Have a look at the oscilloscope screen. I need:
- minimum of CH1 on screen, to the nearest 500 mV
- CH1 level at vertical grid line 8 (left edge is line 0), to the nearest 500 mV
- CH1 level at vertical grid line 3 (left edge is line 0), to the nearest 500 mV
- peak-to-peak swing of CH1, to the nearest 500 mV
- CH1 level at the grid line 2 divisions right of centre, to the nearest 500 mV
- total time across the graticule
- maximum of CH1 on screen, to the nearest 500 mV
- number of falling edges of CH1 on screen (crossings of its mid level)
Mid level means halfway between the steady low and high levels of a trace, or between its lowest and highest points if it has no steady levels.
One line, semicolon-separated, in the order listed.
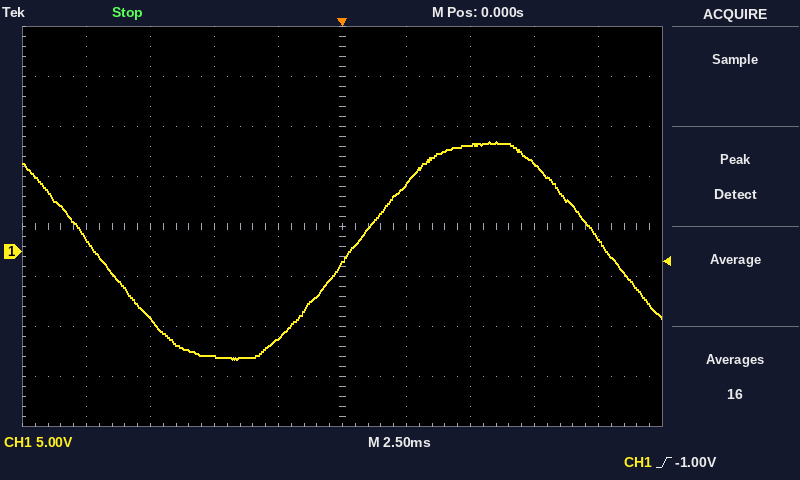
-11.0 V; 9.0 V; -10.5 V; 22.0 V; 10.5 V; 25 ms; 11.0 V; 2
